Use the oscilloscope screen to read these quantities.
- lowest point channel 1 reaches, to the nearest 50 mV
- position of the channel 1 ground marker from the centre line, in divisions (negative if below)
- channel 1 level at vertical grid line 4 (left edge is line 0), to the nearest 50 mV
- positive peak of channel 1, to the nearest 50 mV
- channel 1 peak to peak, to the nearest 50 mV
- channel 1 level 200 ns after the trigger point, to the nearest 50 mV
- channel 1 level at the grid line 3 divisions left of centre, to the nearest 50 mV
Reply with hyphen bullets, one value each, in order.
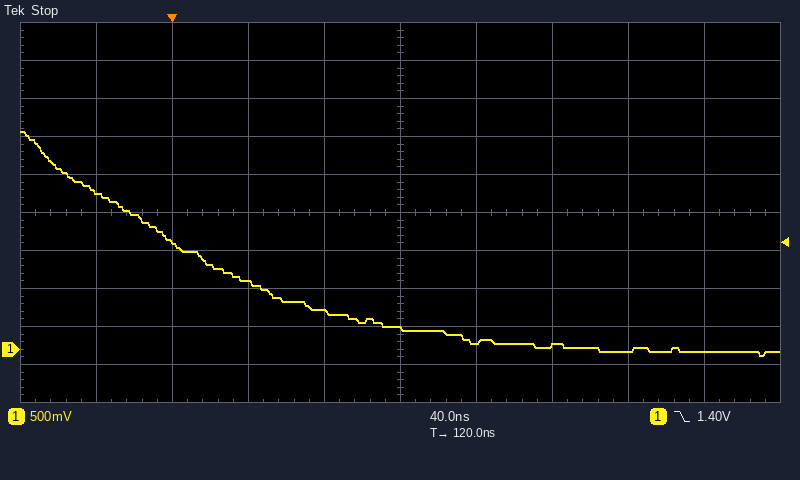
- -100 mV
- -3.6 div
- 500 mV
- 2.85 V
- 2.95 V
- 50 mV
- 1.40 V
